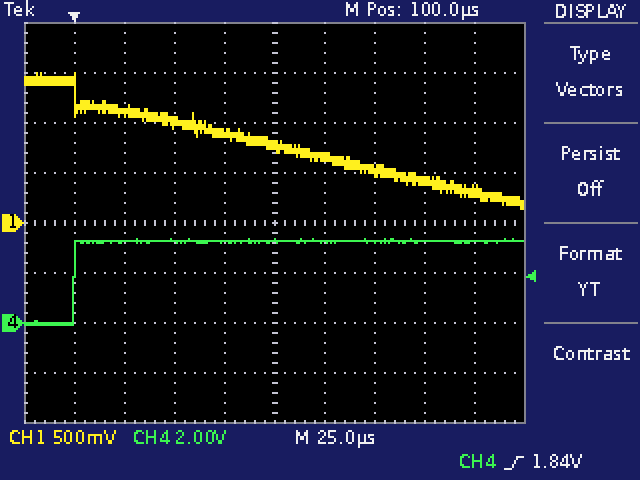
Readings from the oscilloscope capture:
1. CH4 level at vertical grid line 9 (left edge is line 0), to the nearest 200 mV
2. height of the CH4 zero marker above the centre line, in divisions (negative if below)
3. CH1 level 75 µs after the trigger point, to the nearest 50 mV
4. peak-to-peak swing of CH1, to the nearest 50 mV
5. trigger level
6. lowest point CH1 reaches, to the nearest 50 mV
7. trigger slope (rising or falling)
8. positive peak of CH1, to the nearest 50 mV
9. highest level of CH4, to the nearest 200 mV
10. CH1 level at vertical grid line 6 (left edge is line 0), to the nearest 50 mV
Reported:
3.2 V
-2.0 div
900 mV
1.35 V
1.84 V
150 mV
rising
1.50 V
3.4 V
650 mV
